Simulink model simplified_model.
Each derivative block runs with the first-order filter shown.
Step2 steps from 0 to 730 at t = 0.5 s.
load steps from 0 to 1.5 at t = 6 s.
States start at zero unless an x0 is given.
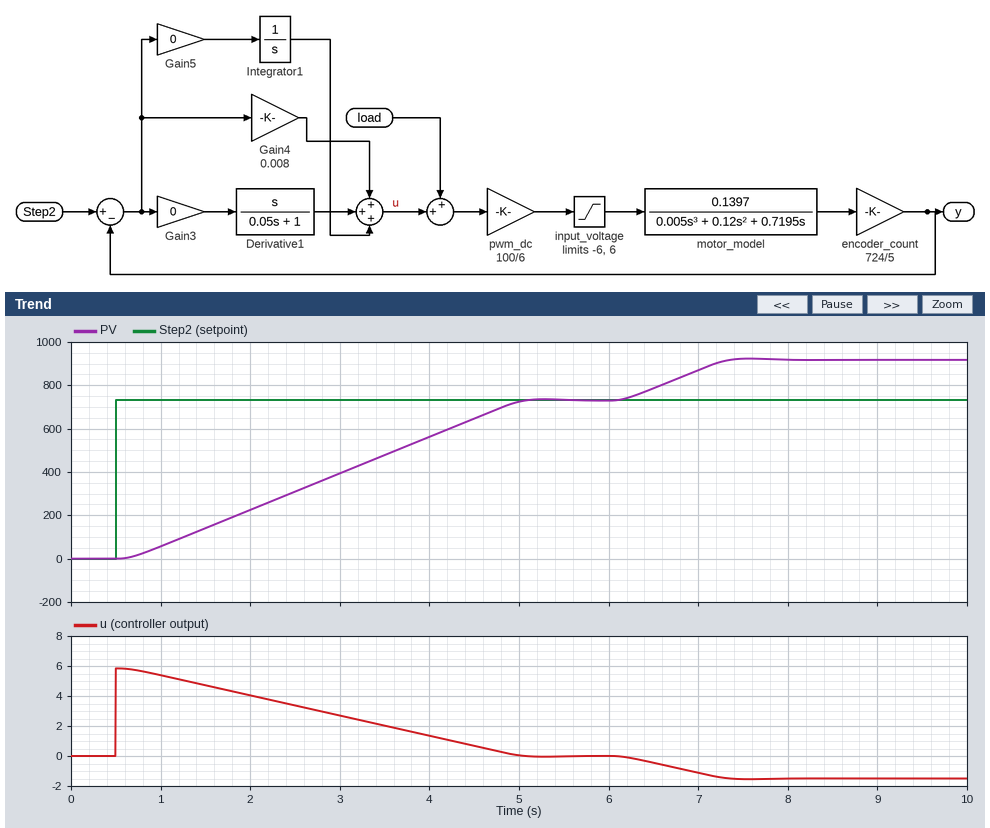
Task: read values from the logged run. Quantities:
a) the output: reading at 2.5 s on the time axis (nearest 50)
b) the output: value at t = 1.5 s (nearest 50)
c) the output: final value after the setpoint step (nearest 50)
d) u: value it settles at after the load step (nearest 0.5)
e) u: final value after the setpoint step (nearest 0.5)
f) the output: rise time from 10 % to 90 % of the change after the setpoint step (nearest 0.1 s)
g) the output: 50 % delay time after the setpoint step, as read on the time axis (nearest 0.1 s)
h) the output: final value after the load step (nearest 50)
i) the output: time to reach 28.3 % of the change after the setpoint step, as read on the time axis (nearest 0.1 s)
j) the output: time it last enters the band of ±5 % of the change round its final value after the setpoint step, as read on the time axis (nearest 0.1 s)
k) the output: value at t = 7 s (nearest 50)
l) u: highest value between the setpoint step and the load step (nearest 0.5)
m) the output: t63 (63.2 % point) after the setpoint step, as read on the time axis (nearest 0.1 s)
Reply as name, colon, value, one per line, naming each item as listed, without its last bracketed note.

the output: reading at 2.5 s on the time axis: 300
the output: value at t = 1.5 s: 150
the output: final value after the setpoint step: 750
u: value it settles at after the load step: -1.5
u: final value after the setpoint step: 0.0
the output: rise time from 10 % to 90 % of the change after the setpoint step: 3.5 s
the output: 50 % delay time after the setpoint step, as read on the time axis: 2.8 s
the output: final value after the load step: 900
the output: time to reach 28.3 % of the change after the setpoint step, as read on the time axis: 1.9 s
the output: time it last enters the band of ±5 % of the change round its final value after the setpoint step, as read on the time axis: 4.8 s
the output: value at t = 7 s: 850
u: highest value between the setpoint step and the load step: 6.0
the output: t63 (63.2 % point) after the setpoint step, as read on the time axis: 3.4 s
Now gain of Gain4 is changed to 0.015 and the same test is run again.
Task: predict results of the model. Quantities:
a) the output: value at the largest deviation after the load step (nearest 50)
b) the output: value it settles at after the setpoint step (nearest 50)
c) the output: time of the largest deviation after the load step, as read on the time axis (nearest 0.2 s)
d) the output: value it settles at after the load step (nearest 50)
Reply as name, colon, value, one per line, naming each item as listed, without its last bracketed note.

the output: value at the largest deviation after the load step: 850
the output: value it settles at after the setpoint step: 750
the output: time of the largest deviation after the load step, as read on the time axis: 7.0 s
the output: value it settles at after the load step: 850
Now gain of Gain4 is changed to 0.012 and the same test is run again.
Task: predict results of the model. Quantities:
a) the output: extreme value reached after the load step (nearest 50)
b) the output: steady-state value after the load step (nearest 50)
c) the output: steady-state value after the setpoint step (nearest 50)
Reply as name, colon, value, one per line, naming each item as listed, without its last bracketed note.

the output: extreme value reached after the load step: 850
the output: steady-state value after the load step: 850
the output: steady-state value after the setpoint step: 750
